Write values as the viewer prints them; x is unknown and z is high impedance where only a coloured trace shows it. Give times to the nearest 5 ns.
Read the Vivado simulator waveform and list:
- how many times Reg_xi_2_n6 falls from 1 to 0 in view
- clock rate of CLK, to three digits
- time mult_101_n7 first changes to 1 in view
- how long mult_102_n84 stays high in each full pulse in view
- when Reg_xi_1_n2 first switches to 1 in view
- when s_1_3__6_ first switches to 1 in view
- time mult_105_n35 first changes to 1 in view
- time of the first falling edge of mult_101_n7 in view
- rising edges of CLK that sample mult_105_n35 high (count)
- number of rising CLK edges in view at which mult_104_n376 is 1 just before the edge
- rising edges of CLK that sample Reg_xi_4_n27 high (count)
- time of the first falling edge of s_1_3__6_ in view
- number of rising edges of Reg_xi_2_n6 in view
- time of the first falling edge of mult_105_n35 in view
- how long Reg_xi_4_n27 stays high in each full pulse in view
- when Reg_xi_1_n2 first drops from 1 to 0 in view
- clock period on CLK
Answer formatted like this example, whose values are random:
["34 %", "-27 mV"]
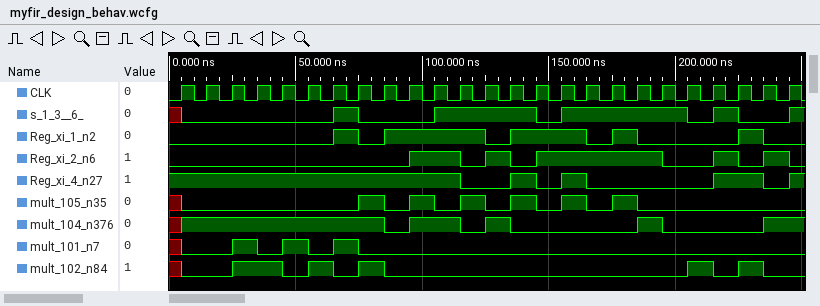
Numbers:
["5", "100 MHz", "25 ns", "20 ns, 10 ns, 10 ns, 10 ns, 10 ns", "65 ns", "65 ns", "75 ns", "35 ns", "6", "13", "16", "75 ns", "5", "85 ns", "10 ns, 10 ns, 20 ns", "75 ns", "10 ns"]
